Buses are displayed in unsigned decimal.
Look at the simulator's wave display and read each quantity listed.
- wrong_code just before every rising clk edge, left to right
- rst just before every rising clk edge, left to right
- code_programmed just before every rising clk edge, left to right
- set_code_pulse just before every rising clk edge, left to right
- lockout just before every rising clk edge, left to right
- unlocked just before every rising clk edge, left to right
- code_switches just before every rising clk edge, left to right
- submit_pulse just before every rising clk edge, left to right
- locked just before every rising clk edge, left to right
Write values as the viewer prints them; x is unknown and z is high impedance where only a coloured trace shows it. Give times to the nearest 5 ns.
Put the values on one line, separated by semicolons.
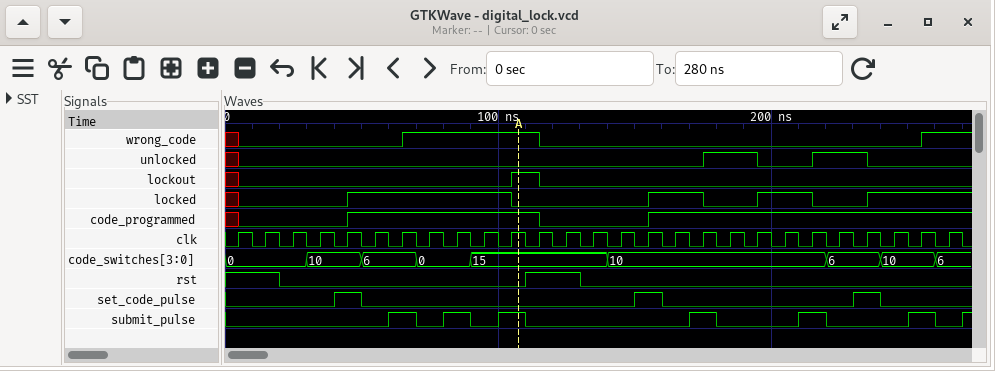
x 0 0 0 0 0 0 1 1 1 1 1 0 0 0 0 0 0 0 0 0 0 0 0 0 0 1; 1 1 0 0 0 0 0 0 0 0 0 1 1 0 0 0 0 0 0 0 0 0 0 0 0 0 0; x 0 0 0 0 1 1 1 1 1 1 1 0 0 0 0 1 1 1 1 1 1 1 1 1 1 1; 0 0 0 0 1 0 0 0 0 0 0 0 0 0 0 1 0 0 0 0 0 0 0 1 0 0 0; x 0 0 0 0 0 0 0 0 0 0 1 0 0 0 0 0 0 0 0 0 0 0 0 0 0 0; x 0 0 0 0 0 0 0 0 0 0 0 0 0 0 0 0 0 1 1 0 0 1 1 0 0 0; 0, 0, 0, 10, 10, 6, 6, 0, 0, 15, 15, 15, 15, 15, 10, 10, 10, 10, 10, 10, 10, 10, 6, 6, 10, 10, 6; 0 0 0 0 0 0 1 0 1 0 1 0 0 0 0 0 0 1 0 0 0 1 0 0 0 1 0; x 0 0 0 0 1 1 1 1 1 1 0 0 0 0 0 1 1 0 0 1 1 0 0 1 1 1
